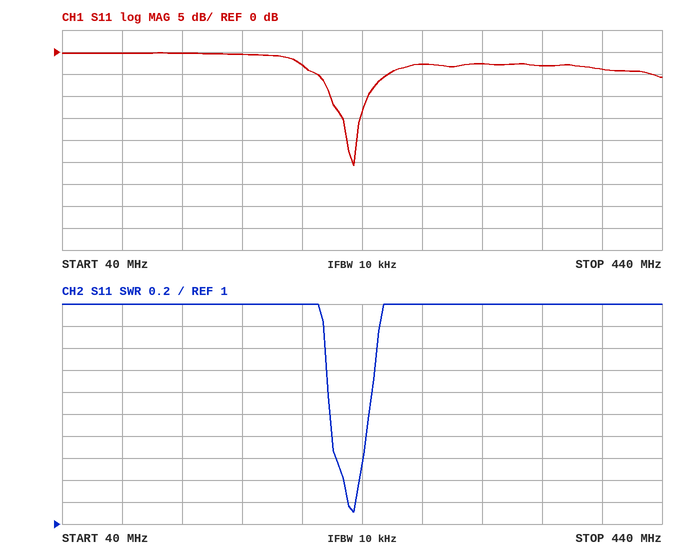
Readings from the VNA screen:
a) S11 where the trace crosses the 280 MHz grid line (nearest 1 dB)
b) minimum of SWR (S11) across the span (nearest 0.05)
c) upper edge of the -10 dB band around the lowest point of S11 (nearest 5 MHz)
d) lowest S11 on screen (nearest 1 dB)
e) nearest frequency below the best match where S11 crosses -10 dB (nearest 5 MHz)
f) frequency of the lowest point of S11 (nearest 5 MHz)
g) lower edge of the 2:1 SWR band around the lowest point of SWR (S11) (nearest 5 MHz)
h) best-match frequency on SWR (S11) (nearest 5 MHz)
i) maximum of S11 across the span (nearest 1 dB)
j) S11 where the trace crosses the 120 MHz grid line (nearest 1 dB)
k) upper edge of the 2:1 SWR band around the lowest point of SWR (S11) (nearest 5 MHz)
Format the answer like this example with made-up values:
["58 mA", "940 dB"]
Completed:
["-3 dB", "1.10", "245 MHz", "-26 dB", "220 MHz", "235 MHz", "220 MHz", "235 MHz", "0 dB", "0 dB", "245 MHz"]
